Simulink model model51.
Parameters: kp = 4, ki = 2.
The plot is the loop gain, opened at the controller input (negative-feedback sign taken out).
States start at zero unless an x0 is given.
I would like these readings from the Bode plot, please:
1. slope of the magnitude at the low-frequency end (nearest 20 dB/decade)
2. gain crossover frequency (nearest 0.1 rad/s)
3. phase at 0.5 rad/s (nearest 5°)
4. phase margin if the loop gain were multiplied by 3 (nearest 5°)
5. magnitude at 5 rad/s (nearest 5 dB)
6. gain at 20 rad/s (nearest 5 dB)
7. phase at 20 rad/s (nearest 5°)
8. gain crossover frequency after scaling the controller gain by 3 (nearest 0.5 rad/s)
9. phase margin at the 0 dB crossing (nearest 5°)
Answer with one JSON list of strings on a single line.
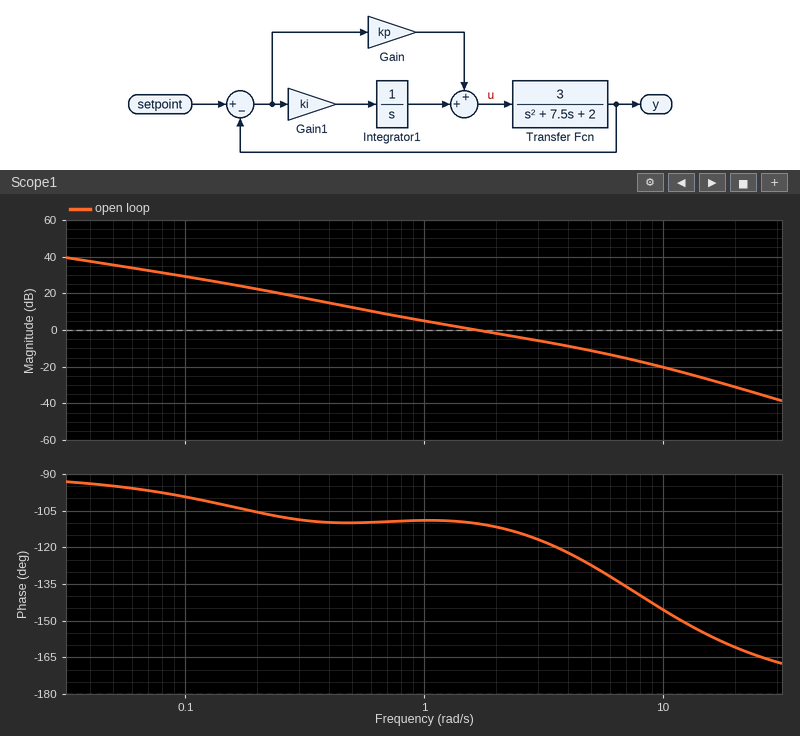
["-20 dB/decade", "1.7 rad/s", "-110°", "55°", "-10 dB", "-30 dB", "-160°", "4.5 rad/s", "70°"]
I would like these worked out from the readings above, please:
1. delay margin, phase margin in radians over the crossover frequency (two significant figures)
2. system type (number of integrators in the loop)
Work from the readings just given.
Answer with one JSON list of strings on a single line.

["0.72 s", "1"]
